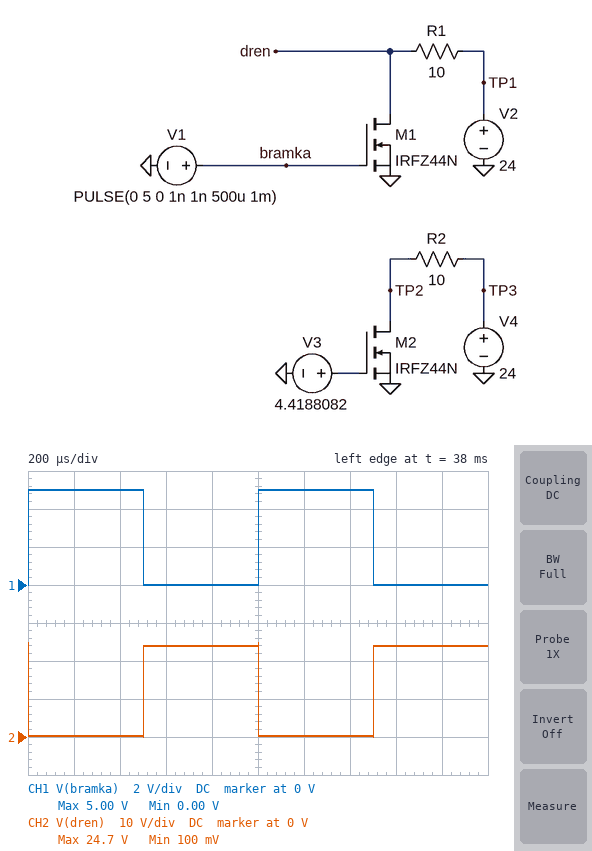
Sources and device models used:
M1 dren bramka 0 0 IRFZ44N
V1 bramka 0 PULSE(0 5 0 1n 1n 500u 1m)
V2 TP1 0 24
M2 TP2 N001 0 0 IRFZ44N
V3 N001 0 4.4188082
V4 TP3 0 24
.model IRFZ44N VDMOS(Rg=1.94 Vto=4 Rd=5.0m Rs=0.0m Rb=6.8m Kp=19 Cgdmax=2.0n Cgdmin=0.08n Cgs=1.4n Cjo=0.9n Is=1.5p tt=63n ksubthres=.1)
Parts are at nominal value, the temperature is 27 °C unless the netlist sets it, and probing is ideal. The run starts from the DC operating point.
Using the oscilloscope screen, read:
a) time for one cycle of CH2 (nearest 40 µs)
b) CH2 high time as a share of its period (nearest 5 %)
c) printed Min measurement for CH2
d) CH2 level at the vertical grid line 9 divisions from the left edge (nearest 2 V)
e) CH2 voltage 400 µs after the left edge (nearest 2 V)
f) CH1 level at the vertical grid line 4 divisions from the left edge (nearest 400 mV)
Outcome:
1.00 ms
50 %
100 mV
24 V
0 V
0 V
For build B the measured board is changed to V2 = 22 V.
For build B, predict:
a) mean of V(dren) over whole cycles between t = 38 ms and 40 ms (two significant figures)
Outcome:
11 V
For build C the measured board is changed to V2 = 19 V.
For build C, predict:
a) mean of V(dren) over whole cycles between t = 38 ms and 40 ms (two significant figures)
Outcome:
9.6 V
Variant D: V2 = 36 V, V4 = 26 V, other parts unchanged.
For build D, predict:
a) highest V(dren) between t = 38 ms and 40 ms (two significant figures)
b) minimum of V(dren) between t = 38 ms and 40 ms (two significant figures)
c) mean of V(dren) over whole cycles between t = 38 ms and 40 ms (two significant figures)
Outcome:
37 V
210 mV
18 V
